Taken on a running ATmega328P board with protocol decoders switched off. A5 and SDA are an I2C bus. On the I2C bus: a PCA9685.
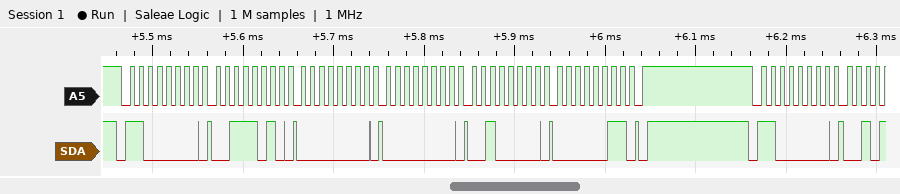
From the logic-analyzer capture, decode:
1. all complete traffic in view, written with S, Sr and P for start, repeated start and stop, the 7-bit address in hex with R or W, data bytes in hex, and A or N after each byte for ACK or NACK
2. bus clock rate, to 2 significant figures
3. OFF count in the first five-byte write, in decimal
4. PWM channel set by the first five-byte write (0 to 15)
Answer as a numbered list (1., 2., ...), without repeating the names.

1. S 60W A 3A A 00 A 00 A 20 A 03 A P S 60W A
2. 100 kHz
3. 800
4. 13
